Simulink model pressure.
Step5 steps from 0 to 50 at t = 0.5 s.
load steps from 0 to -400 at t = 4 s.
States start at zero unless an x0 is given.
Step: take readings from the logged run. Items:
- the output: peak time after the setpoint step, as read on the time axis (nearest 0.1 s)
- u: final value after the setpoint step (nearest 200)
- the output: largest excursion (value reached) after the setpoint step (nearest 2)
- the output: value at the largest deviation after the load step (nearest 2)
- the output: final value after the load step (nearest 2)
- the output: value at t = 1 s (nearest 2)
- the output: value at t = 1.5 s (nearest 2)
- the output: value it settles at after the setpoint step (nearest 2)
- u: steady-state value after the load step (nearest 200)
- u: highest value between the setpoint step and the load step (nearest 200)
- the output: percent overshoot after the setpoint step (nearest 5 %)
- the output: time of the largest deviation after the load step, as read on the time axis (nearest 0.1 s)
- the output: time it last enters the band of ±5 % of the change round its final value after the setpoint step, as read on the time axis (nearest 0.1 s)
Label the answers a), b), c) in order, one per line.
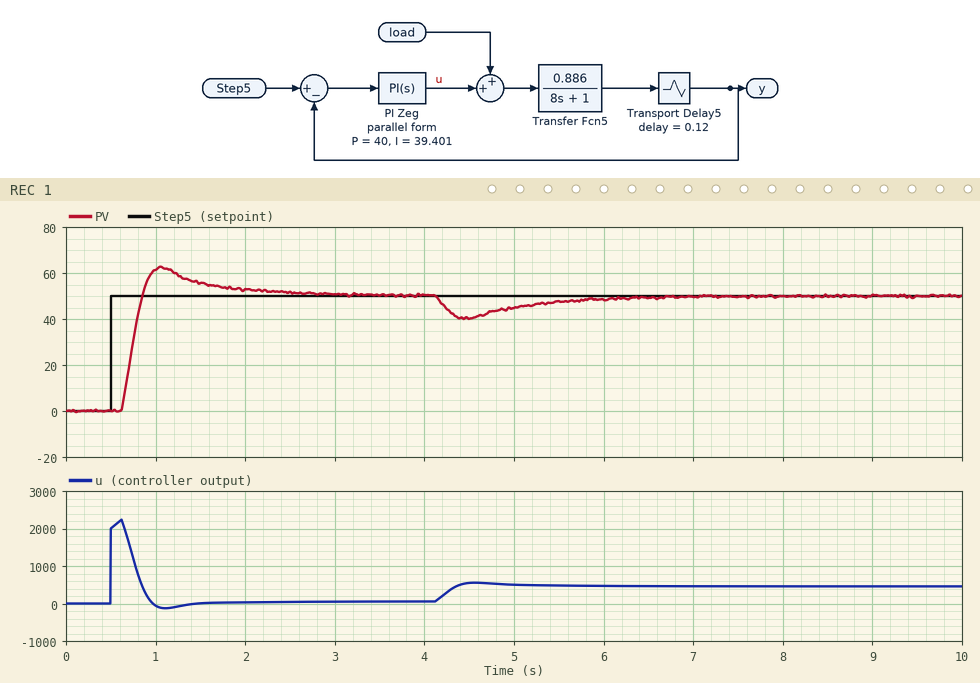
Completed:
a) 1.1 s
b) 0
c) 62
d) 40
e) 50
f) 62
g) 56
h) 50
i) 400
j) 2200
k) 25 %
l) 4.5 s
m) 2.1 s
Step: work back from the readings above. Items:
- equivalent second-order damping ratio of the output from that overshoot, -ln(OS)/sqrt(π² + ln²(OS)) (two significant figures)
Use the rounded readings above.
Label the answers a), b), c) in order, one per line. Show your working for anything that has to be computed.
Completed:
a) ln(0.25) = -1.386; 1.386 / sqrt(9.870 + 1.922) = 0.40
